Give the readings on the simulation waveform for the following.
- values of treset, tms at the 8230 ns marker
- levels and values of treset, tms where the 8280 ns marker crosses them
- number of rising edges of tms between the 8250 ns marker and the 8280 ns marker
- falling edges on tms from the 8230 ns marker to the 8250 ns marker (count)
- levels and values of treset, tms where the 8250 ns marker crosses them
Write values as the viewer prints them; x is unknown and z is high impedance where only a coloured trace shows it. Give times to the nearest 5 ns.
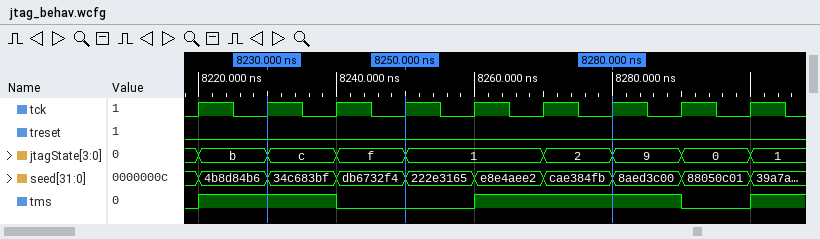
treset=0, tms=1
treset=0, tms=1
1
1
treset=0, tms=0
